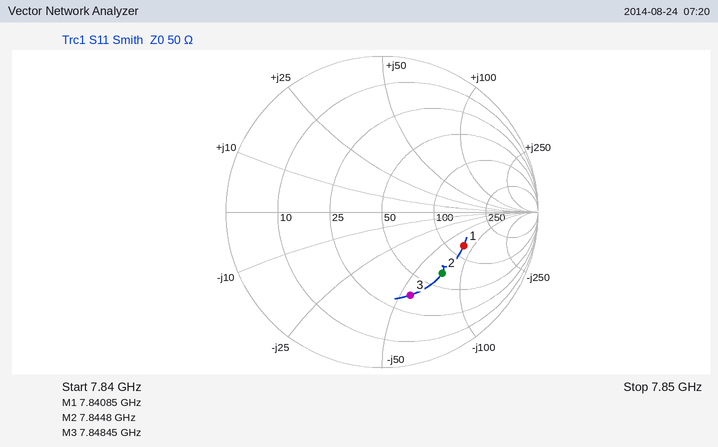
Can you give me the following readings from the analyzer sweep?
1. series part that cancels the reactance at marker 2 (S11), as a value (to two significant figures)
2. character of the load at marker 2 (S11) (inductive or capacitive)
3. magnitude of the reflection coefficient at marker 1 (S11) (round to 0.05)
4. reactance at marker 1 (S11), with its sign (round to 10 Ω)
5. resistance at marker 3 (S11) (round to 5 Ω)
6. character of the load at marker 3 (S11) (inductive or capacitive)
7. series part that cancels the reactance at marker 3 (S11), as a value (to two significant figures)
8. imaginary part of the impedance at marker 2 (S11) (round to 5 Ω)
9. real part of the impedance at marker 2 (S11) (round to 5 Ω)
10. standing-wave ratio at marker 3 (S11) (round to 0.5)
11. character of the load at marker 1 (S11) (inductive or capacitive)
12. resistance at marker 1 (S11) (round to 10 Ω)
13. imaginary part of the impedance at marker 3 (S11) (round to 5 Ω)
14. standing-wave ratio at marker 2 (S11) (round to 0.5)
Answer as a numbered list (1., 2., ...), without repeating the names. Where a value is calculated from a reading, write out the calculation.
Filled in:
1. L = 75 Ω/(2π × 7.8448 GHz) ≈ 1.5 nH
2. capacitive
3. 0.55
4. -80 Ω
5. 35 Ω
6. capacitive
7. L = 55 Ω/(2π × 7.84845 GHz) ≈ 1.1 nH
8. -75 Ω
9. 65 Ω
10. 3.5
11. capacitive
12. 120 Ω
13. -55 Ω
14. 3.5
